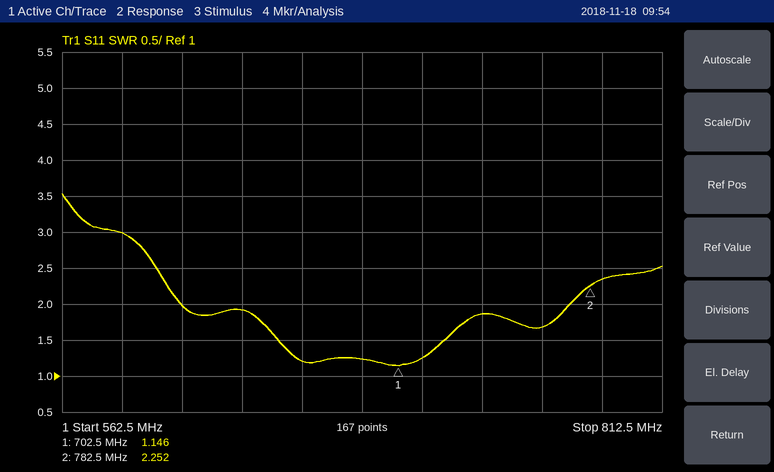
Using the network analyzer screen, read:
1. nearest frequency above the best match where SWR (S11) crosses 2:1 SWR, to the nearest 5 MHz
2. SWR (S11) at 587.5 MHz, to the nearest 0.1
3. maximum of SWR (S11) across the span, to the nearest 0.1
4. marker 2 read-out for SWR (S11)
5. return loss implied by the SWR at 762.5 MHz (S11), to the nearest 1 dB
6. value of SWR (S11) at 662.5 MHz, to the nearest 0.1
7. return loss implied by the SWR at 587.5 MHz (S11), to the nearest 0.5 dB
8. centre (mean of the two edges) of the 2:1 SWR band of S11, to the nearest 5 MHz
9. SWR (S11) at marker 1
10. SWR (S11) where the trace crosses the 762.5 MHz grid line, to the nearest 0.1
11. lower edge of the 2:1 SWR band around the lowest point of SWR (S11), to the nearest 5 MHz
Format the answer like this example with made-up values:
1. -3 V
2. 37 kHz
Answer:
1. 775 MHz
2. 3.0
3. 3.5
4. 2.252
5. 12 dB
6. 1.2
7. 6.0 dB
8. 695 MHz
9. 1.146
10. 1.7
11. 610 MHz
